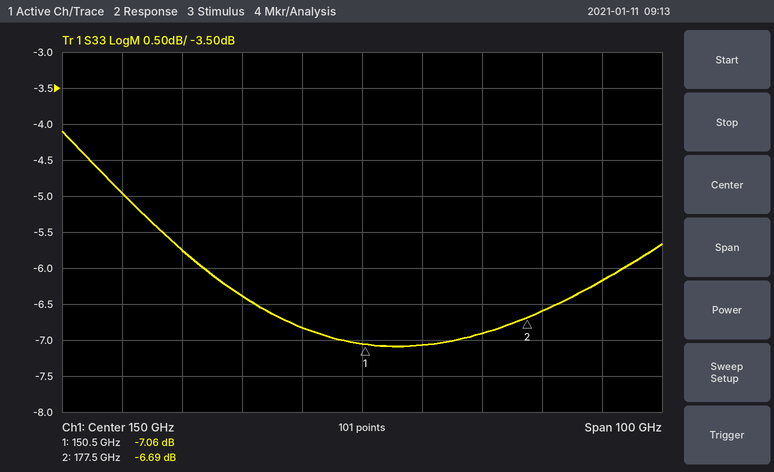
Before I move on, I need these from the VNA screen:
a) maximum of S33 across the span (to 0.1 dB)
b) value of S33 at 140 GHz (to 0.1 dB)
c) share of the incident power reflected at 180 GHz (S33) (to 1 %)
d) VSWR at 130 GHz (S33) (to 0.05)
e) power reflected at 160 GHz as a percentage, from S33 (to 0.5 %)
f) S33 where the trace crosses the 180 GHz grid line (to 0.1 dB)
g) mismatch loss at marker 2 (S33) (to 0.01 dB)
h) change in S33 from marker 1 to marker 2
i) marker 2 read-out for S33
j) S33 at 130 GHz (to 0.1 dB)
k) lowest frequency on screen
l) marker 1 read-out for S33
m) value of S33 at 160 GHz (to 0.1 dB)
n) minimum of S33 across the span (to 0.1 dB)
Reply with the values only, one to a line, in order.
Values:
-4.1 dB
-6.8 dB
22 %
2.85
19.5 %
-6.6 dB
1.05 dB
0.37 dB
-6.69 dB
-6.4 dB
100 GHz
-7.06 dB
-7.1 dB
-7.1 dB
